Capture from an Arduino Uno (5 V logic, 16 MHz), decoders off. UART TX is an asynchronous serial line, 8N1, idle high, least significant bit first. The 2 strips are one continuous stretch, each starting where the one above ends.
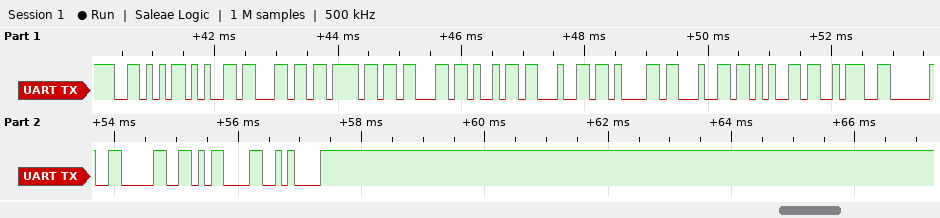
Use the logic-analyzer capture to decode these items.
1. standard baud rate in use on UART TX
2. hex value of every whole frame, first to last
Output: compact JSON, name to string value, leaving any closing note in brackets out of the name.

{"standard baud rate in use on UART TX": "9600 baud", "hex value of every whole frame, first to last": "0x56 0x65 0x6C 0x6F 0x63 0x69 0x64 0x61 0x64 0x65 0x3A 0x20 0x30 0x0D 0x0A"}
